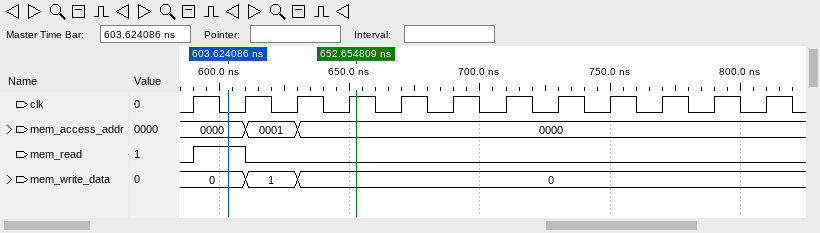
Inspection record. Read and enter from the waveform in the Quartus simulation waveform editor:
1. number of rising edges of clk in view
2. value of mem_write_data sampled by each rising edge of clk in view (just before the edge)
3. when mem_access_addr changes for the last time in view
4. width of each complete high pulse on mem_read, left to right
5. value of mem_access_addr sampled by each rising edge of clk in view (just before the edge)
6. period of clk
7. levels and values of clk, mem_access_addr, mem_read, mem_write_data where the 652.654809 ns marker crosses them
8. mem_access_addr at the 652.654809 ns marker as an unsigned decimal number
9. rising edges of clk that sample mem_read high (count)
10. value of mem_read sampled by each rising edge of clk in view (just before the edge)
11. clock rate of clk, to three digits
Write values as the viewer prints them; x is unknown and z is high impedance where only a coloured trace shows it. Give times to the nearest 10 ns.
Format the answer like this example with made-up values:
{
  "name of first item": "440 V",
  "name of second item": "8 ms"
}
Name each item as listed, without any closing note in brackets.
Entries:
{
  "number of rising edges of clk in view": "12",
  "value of mem_write_data sampled by each rising edge of clk in view": "0, 0, 1, 0, 0, 0, 0, 0, 0, 0, 0, 0",
  "when mem_access_addr changes for the last time in view": "630 ns",
  "width of each complete high pulse on mem_read, left to right": "20 ns",
  "value of mem_access_addr sampled by each rising edge of clk in view": "0000, 0000, 0001, 0000, 0000, 0000, 0000, 0000, 0000, 0000, 0000, 0000",
  "period of clk": "20 ns",
  "levels and values of clk, mem_access_addr, mem_read, mem_write_data where the 652.654809 ns marker crosses them": "clk=1, mem_access_addr=0000, mem_read=0, mem_write_data=0",
  "mem_access_addr at the 652.654809 ns marker as an unsigned decimal number": "0",
  "rising edges of clk that sample mem_read high": "1",
  "value of mem_read sampled by each rising edge of clk in view": "0 1 0 0 0 0 0 0 0 0 0 0",
  "clock rate of clk, to three digits": "50.0 MHz"
}
